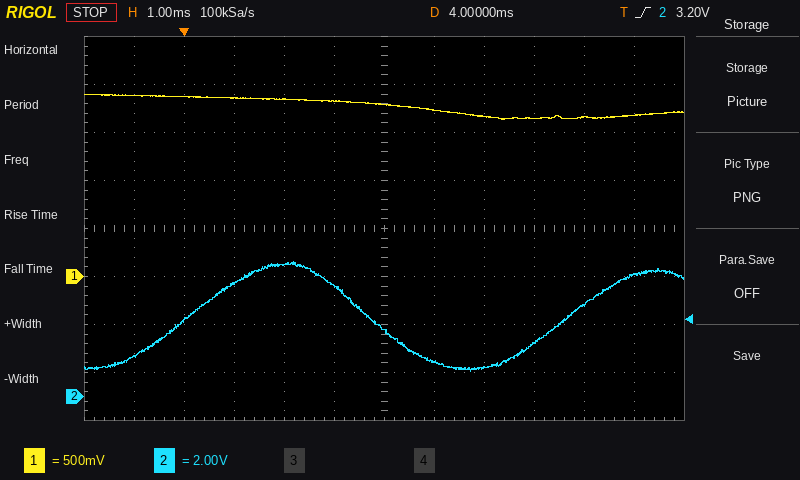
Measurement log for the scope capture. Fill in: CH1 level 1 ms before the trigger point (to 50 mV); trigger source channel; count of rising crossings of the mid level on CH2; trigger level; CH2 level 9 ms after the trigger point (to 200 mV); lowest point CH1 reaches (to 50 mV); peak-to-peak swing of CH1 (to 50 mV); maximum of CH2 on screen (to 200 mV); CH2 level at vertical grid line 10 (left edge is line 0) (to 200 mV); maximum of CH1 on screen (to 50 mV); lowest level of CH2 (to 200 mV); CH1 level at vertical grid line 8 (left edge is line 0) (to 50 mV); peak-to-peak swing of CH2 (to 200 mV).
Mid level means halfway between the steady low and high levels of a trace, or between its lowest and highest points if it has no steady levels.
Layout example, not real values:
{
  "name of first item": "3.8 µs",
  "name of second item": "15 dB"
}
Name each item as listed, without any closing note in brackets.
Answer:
{
  "CH1 level 1 ms before the trigger point": "1.90 V",
  "trigger source channel": "CH2",
  "count of rising crossings of the mid level on CH2": "2",
  "trigger level": "3.20 V",
  "CH2 level 9 ms after the trigger point": "5.0 V",
  "lowest point CH1 reaches": "1.65 V",
  "peak-to-peak swing of CH1": "250 mV",
  "maximum of CH2 on screen": "5.6 V",
  "CH2 level at vertical grid line 10 (left edge is line 0)": "3.8 V",
  "maximum of CH1 on screen": "1.90 V",
  "lowest level of CH2": "1.0 V",
  "CH1 level at vertical grid line 8 (left edge is line 0)": "1.65 V",
  "peak-to-peak swing of CH2": "4.6 V"
}
